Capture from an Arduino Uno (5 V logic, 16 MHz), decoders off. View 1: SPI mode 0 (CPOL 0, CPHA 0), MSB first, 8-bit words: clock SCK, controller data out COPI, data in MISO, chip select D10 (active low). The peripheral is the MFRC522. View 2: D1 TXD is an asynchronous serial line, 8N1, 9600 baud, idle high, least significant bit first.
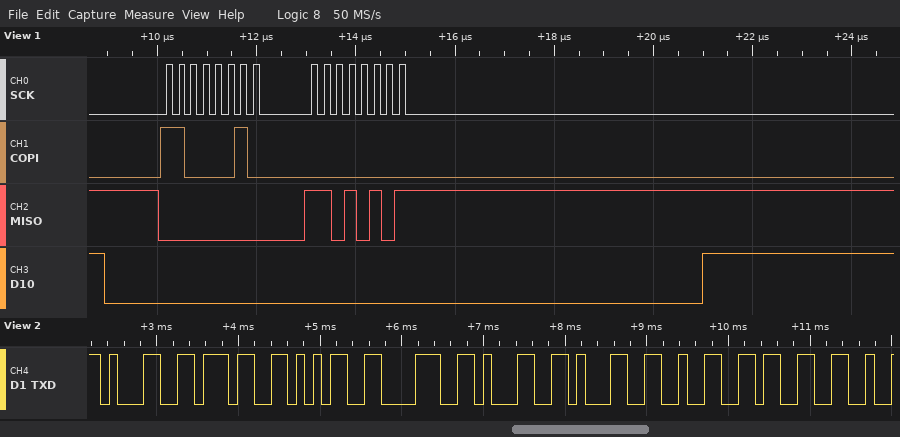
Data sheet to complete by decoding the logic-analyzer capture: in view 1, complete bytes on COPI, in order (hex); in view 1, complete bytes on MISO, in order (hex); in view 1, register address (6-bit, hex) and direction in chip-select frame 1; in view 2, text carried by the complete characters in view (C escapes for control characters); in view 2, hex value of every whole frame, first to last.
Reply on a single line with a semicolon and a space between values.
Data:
C2 00; 00 D5; 0x21 read; "17581123"; 31 37 35 38 31 31 32 33
